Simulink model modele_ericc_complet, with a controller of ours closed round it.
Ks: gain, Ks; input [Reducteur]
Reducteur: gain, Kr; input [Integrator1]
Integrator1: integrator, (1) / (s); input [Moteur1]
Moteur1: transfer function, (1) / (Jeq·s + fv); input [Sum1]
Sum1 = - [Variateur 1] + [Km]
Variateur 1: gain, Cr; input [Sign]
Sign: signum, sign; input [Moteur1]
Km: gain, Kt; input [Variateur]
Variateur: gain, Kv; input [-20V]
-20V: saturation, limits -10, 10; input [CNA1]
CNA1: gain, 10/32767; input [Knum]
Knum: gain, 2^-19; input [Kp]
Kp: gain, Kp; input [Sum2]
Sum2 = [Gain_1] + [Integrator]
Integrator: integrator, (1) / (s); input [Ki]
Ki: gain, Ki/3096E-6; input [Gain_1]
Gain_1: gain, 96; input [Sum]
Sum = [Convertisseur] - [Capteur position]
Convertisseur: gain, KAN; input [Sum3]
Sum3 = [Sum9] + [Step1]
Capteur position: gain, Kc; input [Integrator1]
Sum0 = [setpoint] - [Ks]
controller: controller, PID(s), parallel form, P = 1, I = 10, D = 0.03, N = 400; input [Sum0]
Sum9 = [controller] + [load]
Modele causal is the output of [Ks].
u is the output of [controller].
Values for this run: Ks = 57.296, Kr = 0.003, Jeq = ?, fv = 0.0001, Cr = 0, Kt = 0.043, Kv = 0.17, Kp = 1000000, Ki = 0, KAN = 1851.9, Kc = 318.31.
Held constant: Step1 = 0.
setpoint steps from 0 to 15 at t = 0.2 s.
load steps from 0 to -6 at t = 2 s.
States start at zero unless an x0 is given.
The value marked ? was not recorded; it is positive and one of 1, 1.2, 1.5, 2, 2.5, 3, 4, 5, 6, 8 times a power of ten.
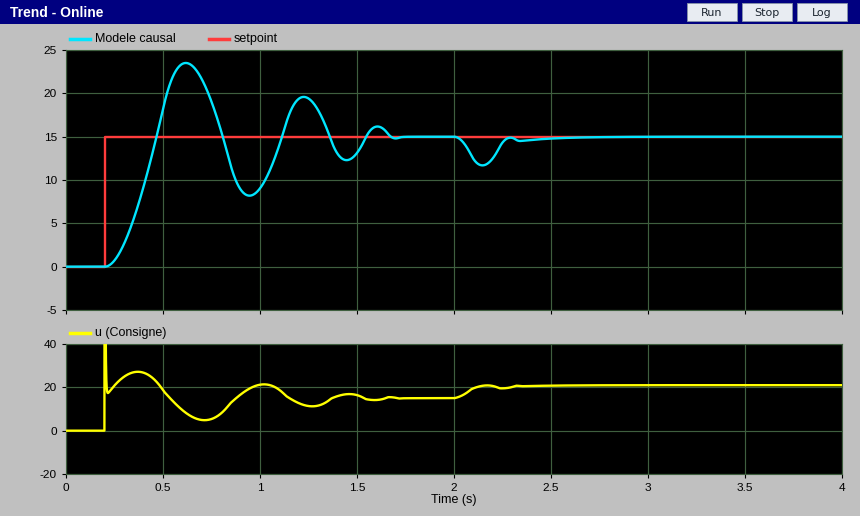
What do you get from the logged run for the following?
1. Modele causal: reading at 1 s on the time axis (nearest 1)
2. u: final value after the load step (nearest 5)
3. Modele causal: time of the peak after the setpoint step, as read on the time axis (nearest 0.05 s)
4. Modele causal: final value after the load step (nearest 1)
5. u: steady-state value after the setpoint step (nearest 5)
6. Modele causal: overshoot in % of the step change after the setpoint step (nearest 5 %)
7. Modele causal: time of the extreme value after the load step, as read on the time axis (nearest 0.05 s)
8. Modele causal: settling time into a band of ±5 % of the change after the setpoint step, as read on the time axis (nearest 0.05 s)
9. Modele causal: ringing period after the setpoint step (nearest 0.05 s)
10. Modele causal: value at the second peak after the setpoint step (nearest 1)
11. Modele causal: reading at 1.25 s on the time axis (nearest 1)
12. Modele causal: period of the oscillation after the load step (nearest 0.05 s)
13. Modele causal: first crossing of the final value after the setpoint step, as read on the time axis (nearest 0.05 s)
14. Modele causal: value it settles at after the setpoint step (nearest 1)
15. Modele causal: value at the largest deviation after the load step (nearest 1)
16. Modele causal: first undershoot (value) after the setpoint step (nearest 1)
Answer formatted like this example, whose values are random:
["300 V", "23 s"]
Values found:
["9", "20", "0.60 s", "15", "15", "55 %", "2.15 s", "1.65 s", "0.60 s", "20", "19", "0.20 s", "0.45 s", "15", "12", "8"]
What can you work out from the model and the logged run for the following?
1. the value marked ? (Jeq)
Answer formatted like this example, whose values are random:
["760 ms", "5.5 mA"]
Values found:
["2e-05"]
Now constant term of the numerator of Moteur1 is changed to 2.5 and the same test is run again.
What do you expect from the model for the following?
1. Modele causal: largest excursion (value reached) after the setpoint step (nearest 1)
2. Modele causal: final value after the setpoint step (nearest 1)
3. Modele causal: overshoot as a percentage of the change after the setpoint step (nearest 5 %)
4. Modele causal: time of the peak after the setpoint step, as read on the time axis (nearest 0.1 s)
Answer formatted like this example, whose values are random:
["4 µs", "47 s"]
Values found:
["19", "15", "25 %", "0.4 s"]
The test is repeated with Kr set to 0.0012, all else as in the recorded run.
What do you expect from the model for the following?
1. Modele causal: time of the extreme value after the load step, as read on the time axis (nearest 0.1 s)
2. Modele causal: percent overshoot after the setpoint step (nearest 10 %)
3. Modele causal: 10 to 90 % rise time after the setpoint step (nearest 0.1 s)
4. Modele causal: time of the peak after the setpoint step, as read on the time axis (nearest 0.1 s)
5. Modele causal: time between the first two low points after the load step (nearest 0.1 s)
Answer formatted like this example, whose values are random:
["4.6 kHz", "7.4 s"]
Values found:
["2.2 s", "30 %", "0.3 s", "0.8 s", "0.3 s"]
